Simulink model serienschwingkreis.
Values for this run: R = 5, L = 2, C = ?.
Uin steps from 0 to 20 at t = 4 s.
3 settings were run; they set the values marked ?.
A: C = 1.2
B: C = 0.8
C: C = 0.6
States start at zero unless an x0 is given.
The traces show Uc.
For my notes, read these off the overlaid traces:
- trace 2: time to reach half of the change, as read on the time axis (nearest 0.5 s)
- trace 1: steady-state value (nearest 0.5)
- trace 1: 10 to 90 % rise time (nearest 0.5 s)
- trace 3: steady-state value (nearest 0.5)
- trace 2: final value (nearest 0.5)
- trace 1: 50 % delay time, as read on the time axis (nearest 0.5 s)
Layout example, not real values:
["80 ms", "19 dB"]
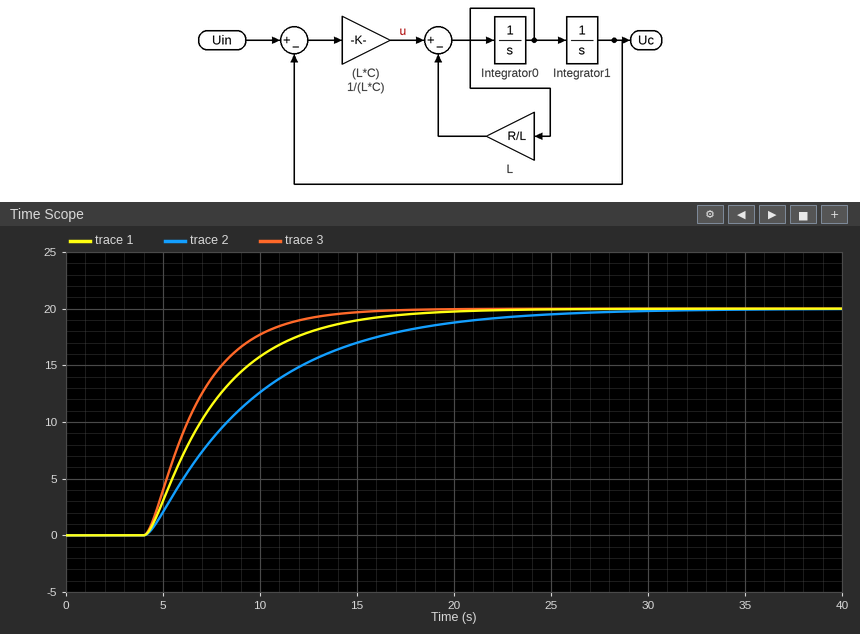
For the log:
["8.5 s", "20.0", "8.0 s", "20.0", "20.0", "7.0 s"]
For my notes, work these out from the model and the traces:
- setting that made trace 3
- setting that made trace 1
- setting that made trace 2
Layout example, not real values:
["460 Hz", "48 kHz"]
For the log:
["C", "B", "A"]
